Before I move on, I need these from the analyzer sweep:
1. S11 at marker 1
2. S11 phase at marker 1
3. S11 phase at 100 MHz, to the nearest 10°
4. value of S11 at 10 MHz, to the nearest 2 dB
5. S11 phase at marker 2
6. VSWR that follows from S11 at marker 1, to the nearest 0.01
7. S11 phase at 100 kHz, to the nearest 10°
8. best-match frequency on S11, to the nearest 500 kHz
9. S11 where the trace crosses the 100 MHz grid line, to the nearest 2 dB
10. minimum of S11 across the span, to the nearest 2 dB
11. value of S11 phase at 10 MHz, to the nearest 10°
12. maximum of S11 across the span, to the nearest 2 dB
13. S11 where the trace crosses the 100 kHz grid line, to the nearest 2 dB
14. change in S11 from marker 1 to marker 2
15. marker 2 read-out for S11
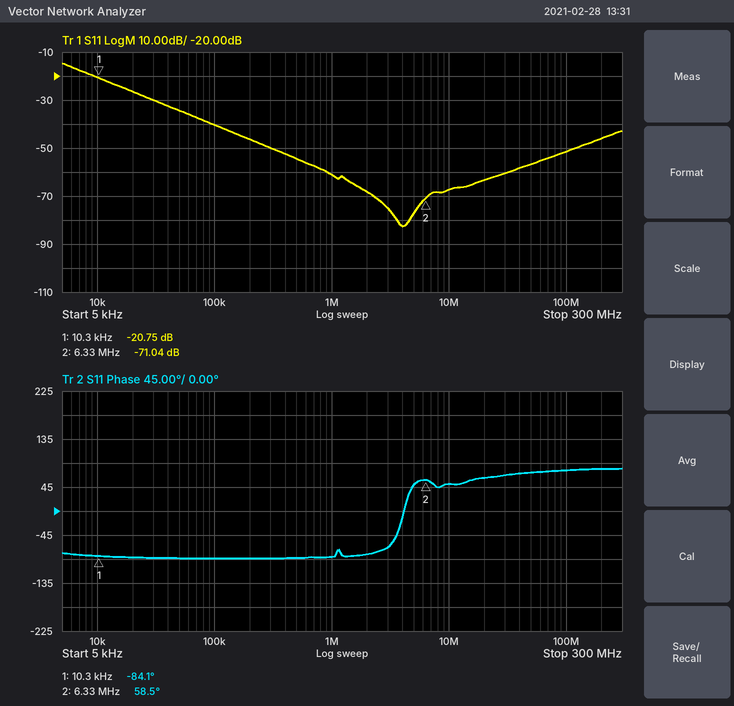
-20.75 dB
-84.1°
80°
-68 dB
58.5°
1.20
-90°
4.0 MHz
-52 dB
-82 dB
50°
-14 dB
-40 dB
-50.29 dB
-71.04 dB
